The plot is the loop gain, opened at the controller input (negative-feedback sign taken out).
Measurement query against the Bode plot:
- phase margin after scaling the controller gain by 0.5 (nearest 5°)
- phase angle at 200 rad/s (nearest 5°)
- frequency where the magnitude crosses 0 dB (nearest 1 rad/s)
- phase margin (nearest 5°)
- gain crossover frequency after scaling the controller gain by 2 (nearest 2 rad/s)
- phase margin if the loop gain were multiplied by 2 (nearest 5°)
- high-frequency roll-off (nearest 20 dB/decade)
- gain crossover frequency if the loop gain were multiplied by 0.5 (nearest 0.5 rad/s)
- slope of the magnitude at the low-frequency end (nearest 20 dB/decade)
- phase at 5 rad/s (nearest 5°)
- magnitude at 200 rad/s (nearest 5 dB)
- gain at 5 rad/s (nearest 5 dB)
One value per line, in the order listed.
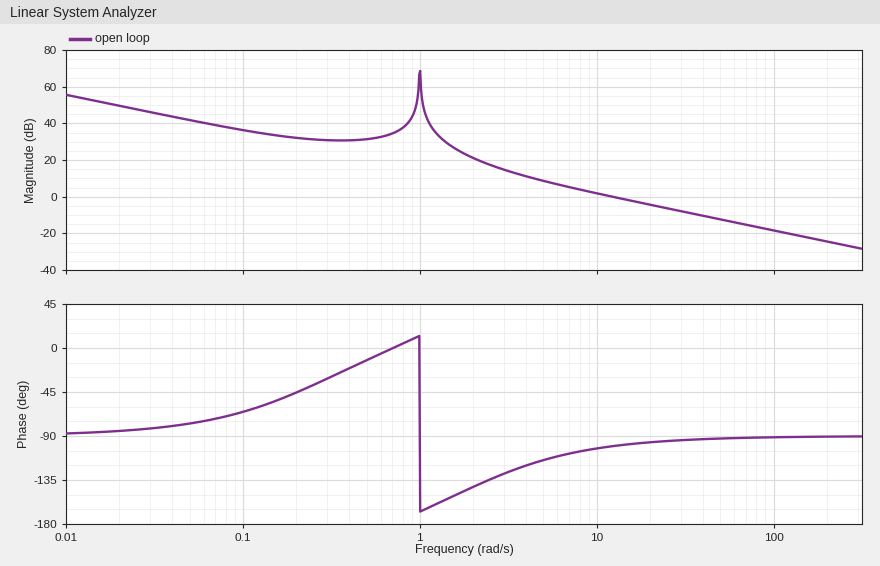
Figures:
70°
-90°
12 rad/s
80°
24 rad/s
85°
-20 dB/decade
6.5 rad/s
-20 dB/decade
-115°
-25 dB
10 dB
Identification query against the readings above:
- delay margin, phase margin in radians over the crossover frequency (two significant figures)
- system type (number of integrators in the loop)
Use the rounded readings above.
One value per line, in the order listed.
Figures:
0.12 s
1
